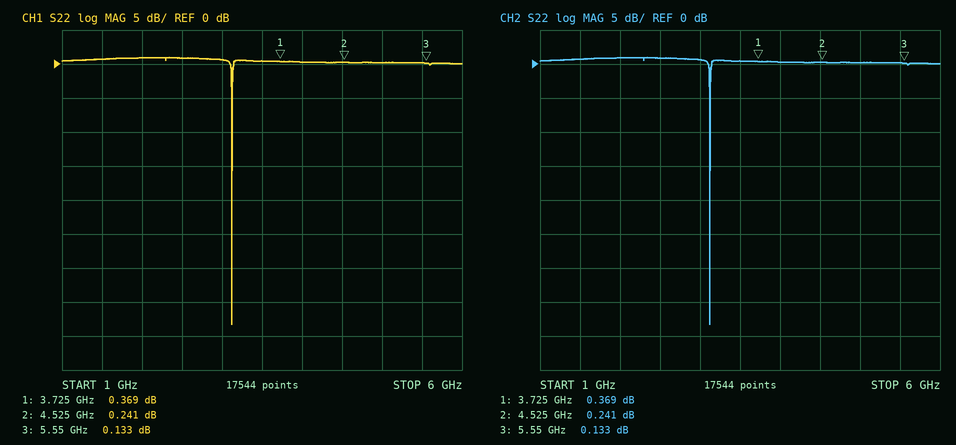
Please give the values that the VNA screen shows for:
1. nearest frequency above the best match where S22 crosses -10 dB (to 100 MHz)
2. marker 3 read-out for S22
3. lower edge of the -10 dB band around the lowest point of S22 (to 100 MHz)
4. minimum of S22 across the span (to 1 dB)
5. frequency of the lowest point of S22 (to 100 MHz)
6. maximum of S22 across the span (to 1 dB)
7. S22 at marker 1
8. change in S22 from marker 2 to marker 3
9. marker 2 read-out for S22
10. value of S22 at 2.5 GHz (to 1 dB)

3.1 GHz
0.133 dB
3.1 GHz
-38 dB
3.1 GHz
1 dB
0.369 dB
-0.108 dB
0.241 dB
1 dB
